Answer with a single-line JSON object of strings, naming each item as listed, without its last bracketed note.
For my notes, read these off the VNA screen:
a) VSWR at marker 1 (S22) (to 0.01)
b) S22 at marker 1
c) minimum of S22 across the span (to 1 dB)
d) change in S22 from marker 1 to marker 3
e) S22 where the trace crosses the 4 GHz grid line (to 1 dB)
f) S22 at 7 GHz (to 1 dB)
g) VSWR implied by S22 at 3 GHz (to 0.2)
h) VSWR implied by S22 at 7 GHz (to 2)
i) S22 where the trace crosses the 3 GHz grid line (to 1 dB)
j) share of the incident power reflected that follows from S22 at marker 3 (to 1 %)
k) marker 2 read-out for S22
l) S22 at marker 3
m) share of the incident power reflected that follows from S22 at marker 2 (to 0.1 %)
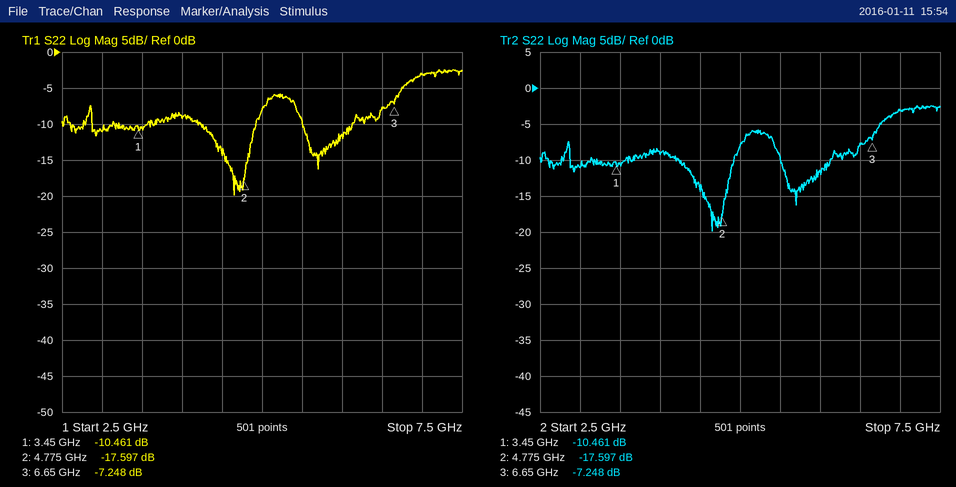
{"VSWR at marker 1 (S22)": "1.86", "S22 at marker 1": "-10.461 dB", "minimum of S22 across the span": "-20 dB", "change in S22 from marker 1 to marker 3": "3.213 dB", "S22 where the trace crosses the 4 GHz grid line": "-9 dB", "S22 at 7 GHz": "-3 dB", "VSWR implied by S22 at 3 GHz": "1.8", "VSWR implied by S22 at 7 GHz": "6", "S22 where the trace crosses the 3 GHz grid line": "-11 dB", "share of the incident power reflected that follows from S22 at marker 3": "19 %", "marker 2 read-out for S22": "-17.597 dB", "S22 at marker 3": "-7.248 dB", "share of the incident power reflected that follows from S22 at marker 2": "1.7 %"}
